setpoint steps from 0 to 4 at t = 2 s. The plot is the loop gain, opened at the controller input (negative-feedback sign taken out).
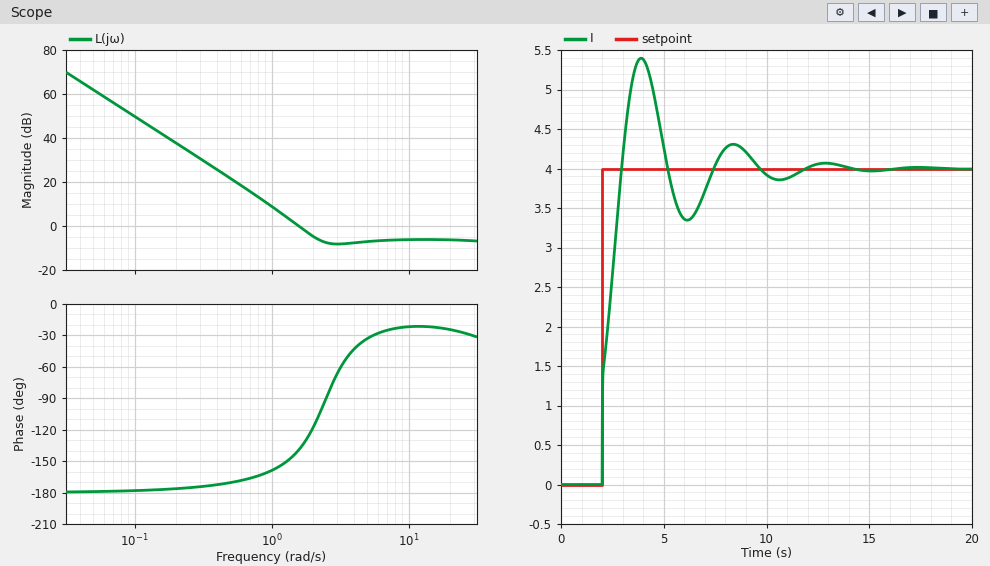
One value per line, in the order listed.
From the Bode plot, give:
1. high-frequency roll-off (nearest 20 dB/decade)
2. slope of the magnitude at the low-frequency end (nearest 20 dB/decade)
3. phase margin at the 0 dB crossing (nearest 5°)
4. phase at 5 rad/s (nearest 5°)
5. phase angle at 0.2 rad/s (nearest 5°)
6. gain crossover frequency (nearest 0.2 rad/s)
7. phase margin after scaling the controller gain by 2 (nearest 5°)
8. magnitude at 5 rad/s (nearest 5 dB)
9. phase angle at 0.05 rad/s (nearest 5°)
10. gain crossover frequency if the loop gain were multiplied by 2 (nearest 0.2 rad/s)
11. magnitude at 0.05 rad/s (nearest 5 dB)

0 dB/decade
-40 dB/decade
40°
-35°
-175°
1.6 rad/s
70°
-5 dB
-180°
2.2 rad/s
60 dB
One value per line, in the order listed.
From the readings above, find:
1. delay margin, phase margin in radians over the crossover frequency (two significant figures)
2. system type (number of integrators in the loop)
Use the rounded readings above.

0.44 s
2
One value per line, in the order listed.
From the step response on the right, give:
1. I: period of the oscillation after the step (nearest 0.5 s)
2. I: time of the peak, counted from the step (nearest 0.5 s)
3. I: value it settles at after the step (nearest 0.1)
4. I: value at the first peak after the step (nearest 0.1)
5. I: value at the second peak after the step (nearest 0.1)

4.5 s
2.0 s
4.0
5.4
4.3
